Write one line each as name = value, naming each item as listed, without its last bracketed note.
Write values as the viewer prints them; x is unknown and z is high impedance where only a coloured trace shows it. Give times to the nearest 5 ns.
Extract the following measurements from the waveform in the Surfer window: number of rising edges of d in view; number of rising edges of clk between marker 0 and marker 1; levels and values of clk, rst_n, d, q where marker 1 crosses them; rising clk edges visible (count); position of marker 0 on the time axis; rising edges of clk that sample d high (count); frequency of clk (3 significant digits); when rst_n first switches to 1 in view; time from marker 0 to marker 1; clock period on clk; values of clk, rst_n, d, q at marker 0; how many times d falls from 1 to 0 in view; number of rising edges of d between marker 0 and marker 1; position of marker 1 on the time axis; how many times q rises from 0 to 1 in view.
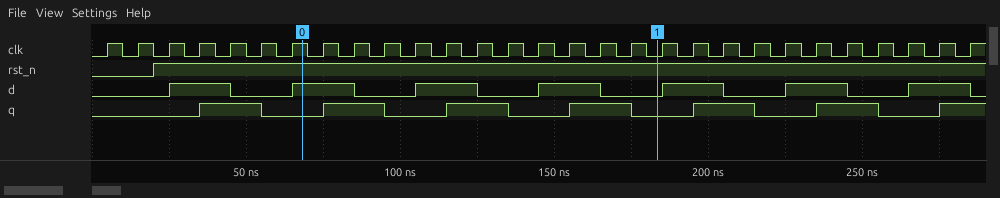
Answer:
number of rising edges of d in view = 7
number of rising edges of clk between marker 0 and marker 1 = 11
levels and values of clk, rst_n, d, q where marker 1 crosses them = clk=0, rst_n=1, d=0, q=0
rising clk edges visible = 29
position of marker 0 on the time axis = 70 ns
rising edges of clk that sample d high = 14
frequency of clk = 100 MHz
when rst_n first switches to 1 in view = 20 ns
time from marker 0 to marker 1 = 115 ns
clock period on clk = 10 ns
values of clk, rst_n, d, q at marker 0 = clk=1, rst_n=1, d=1, q=0
how many times d falls from 1 to 0 in view = 7
number of rising edges of d between marker 0 and marker 1 = 2
position of marker 1 on the time axis = 185 ns
how many times q rises from 0 to 1 in view = 7
